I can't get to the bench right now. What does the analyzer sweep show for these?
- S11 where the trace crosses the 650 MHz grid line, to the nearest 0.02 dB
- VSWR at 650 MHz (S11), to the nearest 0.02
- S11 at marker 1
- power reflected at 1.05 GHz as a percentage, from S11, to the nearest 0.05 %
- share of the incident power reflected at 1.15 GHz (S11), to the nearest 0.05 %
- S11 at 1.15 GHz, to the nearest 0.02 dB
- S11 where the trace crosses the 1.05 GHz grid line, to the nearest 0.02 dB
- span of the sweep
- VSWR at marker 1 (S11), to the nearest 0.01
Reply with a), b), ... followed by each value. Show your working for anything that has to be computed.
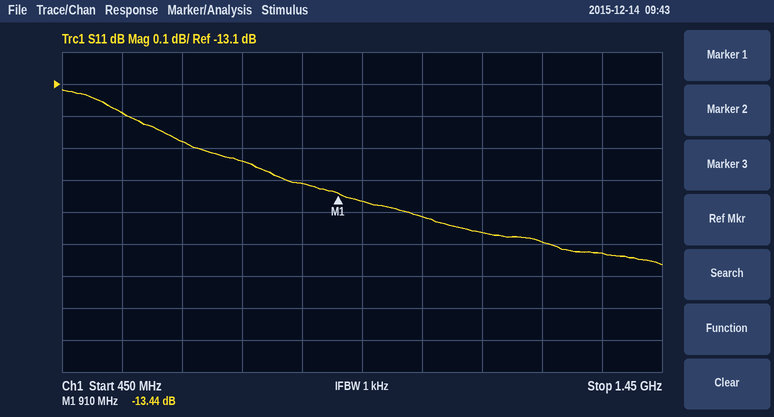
a) -13.28 dB
b) |Γ| = 10^(-13.28/20) = 0.2168; VSWR = (1 + 0.2168)/(1 − 0.2168) ≈ 1.55, so 1.56 to the nearest 0.02
c) -13.44 dB
d) 10^(-13.52/10) ≈ 4.45 %
e) 10^(-13.56/10) ≈ 4.41 %, so 4.40 % to the nearest 0.05 %
f) -13.56 dB
g) -13.52 dB
h) 1 GHz
i) (1 + 0.2128)/(1 − 0.2128) ≈ 1.54
